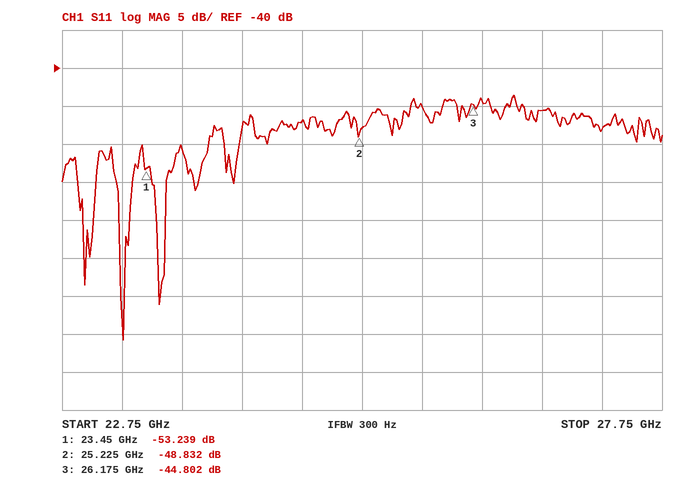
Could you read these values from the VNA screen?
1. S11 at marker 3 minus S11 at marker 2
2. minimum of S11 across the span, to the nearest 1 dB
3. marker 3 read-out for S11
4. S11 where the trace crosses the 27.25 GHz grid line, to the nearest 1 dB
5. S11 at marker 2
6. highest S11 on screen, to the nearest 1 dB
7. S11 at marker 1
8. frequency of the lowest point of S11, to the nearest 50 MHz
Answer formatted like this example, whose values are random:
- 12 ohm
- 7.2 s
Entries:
- 4.030 dB
- -76 dB
- -44.802 dB
- -48 dB
- -48.832 dB
- -44 dB
- -53.239 dB
- 23.25 GHz
